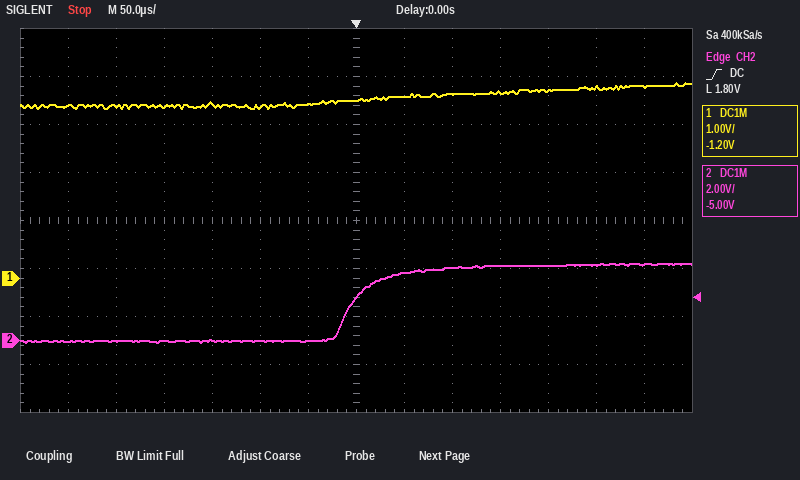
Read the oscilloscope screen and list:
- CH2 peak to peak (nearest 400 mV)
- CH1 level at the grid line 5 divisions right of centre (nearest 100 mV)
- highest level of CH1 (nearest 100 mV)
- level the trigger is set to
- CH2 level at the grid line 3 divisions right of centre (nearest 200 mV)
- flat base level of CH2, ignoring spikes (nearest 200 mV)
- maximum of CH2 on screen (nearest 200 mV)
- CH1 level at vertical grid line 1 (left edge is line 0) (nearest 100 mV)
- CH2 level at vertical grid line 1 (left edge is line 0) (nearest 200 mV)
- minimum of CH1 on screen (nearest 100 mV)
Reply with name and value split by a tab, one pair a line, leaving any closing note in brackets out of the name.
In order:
CH2 peak to peak	3.2 V
CH1 level at the grid line 5 divisions right of centre	4.0 V
highest level of CH1	4.1 V
level the trigger is set to	1.80 V
CH2 level at the grid line 3 divisions right of centre	3.2 V
flat base level of CH2, ignoring spikes	0.0 V
maximum of CH2 on screen	3.2 V
CH1 level at vertical grid line 1 (left edge is line 0)	3.6 V
CH2 level at vertical grid line 1 (left edge is line 0)	0.0 V
minimum of CH1 on screen	3.5 V
